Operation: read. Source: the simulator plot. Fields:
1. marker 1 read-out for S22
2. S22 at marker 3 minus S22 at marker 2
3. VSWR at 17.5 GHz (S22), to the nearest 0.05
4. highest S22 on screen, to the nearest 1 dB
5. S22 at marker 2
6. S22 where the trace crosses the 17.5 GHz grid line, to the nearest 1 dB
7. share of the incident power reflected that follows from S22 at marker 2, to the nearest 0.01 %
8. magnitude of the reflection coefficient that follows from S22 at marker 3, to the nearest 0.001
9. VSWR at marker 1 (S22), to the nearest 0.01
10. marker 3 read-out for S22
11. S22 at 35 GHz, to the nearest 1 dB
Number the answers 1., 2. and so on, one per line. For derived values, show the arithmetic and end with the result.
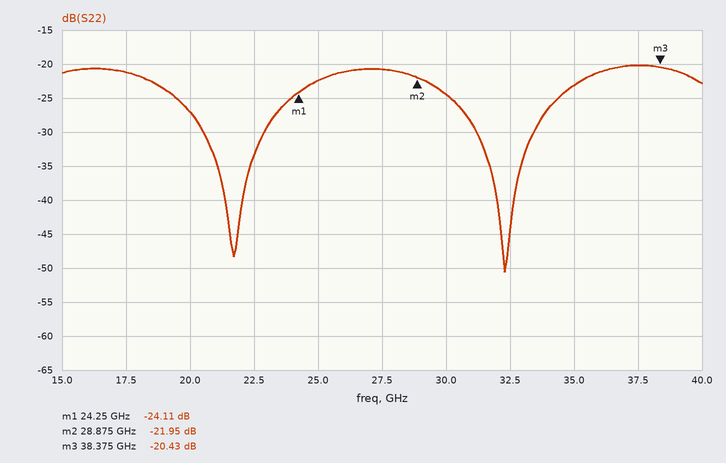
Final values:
1. -24.11 dB
2. -20.43 − (-21.95) = 1.52 dB
3. |Γ| = 10^(-21/20) = 0.0891; VSWR = (1 + 0.0891)/(1 − 0.0891) ≈ 1.20
4. -20 dB
5. -21.95 dB
6. -21 dB
7. 10^(-21.95/10) ≈ 0.64 %
8. 10^(-20.43/20) ≈ 0.095
9. (1 + 0.0623)/(1 − 0.0623) ≈ 1.13
10. -20.43 dB
11. -23 dB
